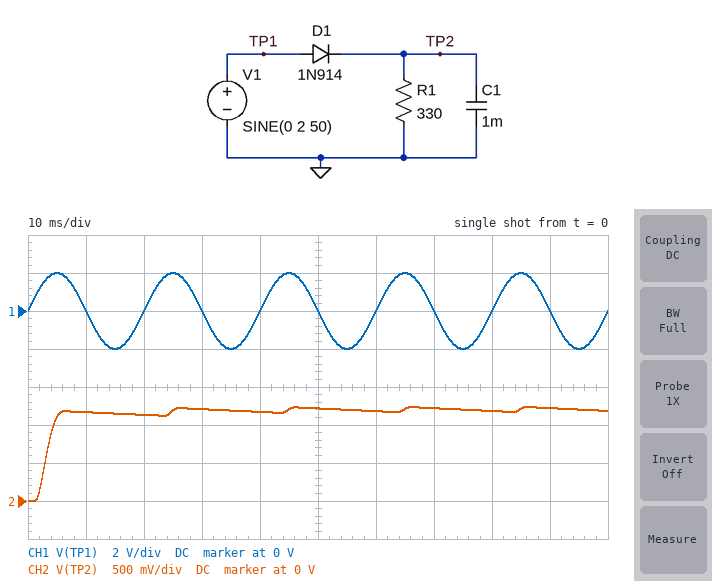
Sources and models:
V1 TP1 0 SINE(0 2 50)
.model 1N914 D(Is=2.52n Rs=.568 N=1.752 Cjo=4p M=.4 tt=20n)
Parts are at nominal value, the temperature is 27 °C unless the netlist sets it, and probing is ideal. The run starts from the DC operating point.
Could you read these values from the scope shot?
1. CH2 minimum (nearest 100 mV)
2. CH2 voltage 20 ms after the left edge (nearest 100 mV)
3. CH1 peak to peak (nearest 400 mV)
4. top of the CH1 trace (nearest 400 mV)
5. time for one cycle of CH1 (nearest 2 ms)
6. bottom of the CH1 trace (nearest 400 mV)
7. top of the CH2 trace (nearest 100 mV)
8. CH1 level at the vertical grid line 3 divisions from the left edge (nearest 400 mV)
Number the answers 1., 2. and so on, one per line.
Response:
1. 0 V
2. 1.1 V
3. 4.0 V
4. 2.0 V
5. 20 ms
6. -2.0 V
7. 1.2 V
8. 0 V
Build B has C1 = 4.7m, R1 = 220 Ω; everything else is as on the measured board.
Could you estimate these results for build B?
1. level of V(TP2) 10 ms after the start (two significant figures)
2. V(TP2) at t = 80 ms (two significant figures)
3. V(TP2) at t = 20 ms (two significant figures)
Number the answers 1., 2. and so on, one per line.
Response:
1. 820 mV
2. 1.1 V
3. 810 mV
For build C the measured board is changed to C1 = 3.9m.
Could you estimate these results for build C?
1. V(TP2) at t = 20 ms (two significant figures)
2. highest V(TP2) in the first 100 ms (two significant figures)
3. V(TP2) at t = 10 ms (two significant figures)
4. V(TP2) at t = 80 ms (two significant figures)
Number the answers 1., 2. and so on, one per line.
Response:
1. 870 mV
2. 1.2 V
3. 880 mV
4. 1.1 V
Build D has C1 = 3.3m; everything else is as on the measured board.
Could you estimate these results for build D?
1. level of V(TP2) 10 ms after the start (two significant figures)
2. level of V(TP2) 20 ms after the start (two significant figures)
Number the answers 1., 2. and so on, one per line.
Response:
1. 930 mV
2. 920 mV
